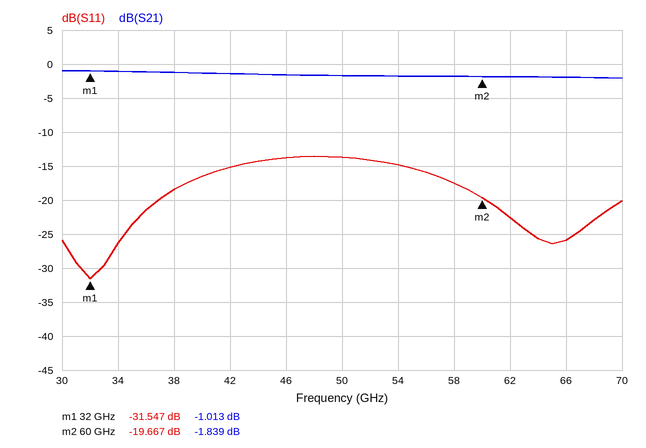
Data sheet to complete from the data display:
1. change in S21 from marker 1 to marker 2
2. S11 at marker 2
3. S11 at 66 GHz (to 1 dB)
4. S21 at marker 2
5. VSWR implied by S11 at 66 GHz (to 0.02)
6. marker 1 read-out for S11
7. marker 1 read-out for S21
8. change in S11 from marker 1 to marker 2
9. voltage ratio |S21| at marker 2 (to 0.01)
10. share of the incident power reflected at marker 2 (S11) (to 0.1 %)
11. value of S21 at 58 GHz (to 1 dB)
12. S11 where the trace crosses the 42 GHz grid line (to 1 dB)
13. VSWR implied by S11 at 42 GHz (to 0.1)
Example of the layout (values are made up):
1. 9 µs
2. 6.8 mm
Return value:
1. -0.826 dB
2. -19.667 dB
3. -26 dB
4. -1.839 dB
5. 1.10
6. -31.547 dB
7. -1.013 dB
8. 11.880 dB
9. 0.81
10. 1.1 %
11. -2 dB
12. -15 dB
13. 1.4
